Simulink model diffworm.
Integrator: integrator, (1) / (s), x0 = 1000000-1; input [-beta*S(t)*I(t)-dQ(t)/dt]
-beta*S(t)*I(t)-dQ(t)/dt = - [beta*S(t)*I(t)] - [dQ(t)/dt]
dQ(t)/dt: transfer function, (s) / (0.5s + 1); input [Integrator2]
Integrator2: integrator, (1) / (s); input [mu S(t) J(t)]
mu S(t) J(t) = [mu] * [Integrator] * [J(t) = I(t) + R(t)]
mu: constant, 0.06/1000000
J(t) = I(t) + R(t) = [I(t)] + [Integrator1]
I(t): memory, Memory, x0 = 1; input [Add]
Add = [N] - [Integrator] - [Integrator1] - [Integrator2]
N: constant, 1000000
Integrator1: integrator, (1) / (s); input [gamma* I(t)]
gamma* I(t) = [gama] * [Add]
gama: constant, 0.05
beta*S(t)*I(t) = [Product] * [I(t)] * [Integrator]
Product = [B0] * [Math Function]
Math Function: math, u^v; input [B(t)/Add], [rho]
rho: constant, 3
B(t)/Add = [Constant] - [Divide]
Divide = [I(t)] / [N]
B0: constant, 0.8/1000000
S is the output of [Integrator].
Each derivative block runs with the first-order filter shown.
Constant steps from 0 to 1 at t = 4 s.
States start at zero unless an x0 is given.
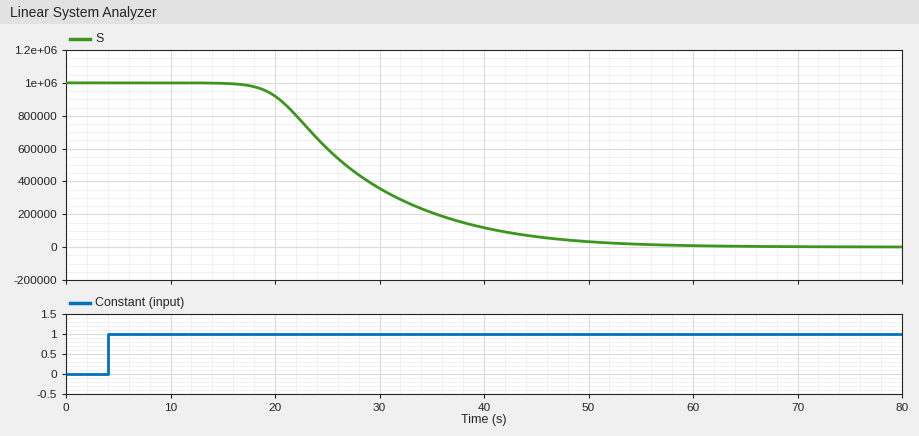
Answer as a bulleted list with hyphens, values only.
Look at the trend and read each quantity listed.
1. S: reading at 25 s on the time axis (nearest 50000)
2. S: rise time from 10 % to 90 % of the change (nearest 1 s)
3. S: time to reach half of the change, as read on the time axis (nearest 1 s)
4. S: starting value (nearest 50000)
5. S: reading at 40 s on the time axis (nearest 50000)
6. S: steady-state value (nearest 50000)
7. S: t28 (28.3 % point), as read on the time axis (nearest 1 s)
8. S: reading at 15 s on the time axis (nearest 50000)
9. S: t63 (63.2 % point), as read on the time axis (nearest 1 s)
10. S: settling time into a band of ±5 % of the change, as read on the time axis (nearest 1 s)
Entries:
- 600000
- 21 s
- 27 s
- 1000000
- 100000
- 0
- 23 s
- 1000000
- 30 s
- 47 s
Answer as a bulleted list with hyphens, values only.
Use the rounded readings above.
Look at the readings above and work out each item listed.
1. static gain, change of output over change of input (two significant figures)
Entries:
- -1000000
